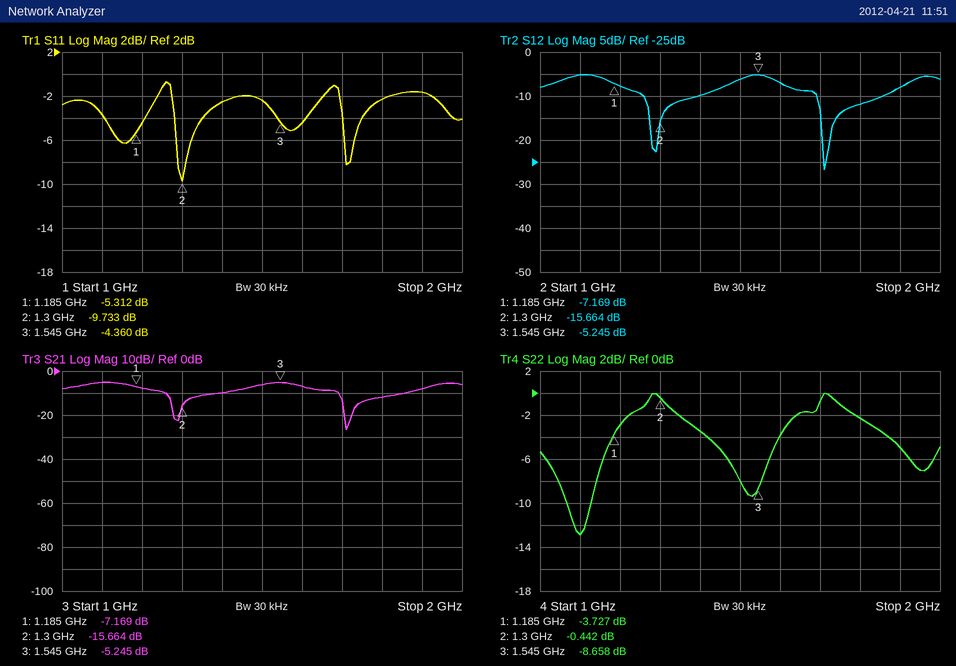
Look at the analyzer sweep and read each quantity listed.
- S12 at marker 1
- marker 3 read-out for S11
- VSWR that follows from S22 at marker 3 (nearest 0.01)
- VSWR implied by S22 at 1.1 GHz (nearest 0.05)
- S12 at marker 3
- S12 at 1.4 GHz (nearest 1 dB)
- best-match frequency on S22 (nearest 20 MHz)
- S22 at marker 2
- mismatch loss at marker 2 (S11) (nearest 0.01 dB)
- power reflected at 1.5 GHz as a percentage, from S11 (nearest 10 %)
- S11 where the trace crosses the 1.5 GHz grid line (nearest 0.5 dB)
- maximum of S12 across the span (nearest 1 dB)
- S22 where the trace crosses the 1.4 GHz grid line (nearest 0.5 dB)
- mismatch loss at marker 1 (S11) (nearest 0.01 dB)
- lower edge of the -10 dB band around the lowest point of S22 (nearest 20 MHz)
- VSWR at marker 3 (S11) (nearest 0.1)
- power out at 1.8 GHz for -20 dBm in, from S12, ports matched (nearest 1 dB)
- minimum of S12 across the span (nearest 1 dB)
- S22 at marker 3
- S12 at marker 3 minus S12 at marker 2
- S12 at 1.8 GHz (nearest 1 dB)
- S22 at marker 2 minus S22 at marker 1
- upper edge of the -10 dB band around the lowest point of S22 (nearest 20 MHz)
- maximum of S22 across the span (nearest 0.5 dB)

-7.169 dB
-4.360 dB
2.17
1.60
-5.245 dB
-10 dB
1.10 GHz
-0.442 dB
0.49 dB
60 %
-2.5 dB
-5 dB
-3.5 dB
1.51 dB
1.06 GHz
4.1
-32 dBm
-27 dB
-8.658 dB
10.419 dB
-12 dB
3.285 dB
1.12 GHz
0.0 dB
